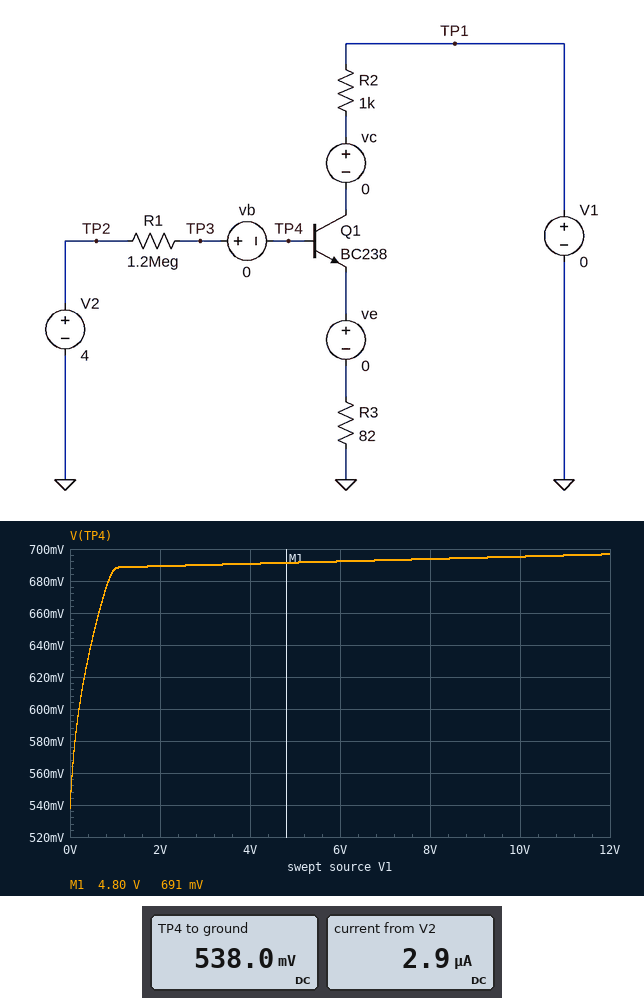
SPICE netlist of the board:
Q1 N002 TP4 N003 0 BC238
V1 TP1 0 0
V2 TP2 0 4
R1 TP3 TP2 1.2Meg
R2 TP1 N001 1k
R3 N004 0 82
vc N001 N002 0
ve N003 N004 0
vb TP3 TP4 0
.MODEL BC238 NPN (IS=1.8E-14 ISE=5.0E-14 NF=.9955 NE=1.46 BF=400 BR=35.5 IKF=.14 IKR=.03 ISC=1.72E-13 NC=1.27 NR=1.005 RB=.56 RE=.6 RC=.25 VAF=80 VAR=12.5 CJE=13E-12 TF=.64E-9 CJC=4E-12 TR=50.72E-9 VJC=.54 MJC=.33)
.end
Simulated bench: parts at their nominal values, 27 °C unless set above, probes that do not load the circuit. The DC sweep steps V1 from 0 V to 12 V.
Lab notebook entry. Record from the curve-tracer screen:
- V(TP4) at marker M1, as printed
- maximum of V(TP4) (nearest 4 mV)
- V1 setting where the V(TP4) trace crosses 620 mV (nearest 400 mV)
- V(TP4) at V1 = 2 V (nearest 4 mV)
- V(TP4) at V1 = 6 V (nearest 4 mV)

691 mV
696 mV
400 mV
688 mV
692 mV
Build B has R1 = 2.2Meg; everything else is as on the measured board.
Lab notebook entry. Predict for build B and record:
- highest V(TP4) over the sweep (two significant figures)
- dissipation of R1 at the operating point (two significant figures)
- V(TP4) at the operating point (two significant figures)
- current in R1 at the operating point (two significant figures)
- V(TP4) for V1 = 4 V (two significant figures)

650 mV
5.5 µW
520 mV
1.6 µA
640 mV
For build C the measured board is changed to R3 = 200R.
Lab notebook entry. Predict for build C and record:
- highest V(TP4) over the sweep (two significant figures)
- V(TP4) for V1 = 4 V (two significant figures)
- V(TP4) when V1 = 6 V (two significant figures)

790 mV
770 mV
780 mV
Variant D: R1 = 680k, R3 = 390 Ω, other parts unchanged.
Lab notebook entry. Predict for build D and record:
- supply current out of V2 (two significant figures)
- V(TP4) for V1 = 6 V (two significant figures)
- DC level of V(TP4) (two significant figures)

5.1 µA
1.1 V
560 mV
